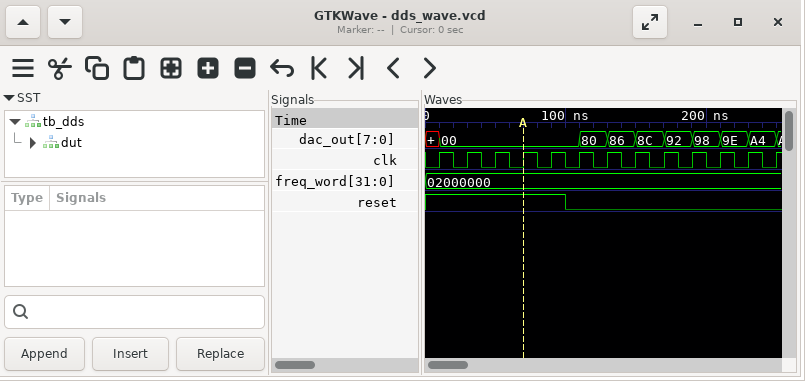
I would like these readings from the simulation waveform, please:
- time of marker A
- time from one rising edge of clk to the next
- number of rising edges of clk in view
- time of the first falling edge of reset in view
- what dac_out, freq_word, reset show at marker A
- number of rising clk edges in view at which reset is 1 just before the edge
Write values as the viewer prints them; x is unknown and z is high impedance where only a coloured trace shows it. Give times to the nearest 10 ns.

70 ns
20 ns
13
100 ns
dac_out=00, freq_word=02000000, reset=1
5
